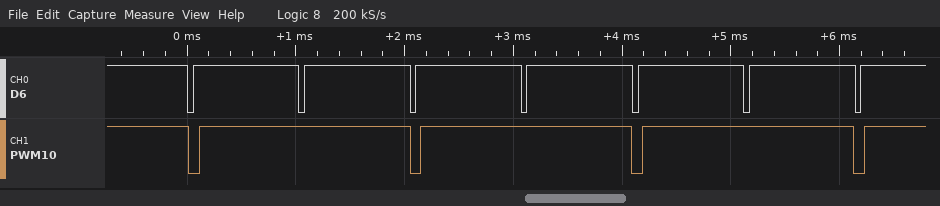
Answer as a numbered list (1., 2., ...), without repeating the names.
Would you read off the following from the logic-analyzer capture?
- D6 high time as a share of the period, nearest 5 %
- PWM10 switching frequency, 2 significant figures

1. 95 %
2. 490 Hz
